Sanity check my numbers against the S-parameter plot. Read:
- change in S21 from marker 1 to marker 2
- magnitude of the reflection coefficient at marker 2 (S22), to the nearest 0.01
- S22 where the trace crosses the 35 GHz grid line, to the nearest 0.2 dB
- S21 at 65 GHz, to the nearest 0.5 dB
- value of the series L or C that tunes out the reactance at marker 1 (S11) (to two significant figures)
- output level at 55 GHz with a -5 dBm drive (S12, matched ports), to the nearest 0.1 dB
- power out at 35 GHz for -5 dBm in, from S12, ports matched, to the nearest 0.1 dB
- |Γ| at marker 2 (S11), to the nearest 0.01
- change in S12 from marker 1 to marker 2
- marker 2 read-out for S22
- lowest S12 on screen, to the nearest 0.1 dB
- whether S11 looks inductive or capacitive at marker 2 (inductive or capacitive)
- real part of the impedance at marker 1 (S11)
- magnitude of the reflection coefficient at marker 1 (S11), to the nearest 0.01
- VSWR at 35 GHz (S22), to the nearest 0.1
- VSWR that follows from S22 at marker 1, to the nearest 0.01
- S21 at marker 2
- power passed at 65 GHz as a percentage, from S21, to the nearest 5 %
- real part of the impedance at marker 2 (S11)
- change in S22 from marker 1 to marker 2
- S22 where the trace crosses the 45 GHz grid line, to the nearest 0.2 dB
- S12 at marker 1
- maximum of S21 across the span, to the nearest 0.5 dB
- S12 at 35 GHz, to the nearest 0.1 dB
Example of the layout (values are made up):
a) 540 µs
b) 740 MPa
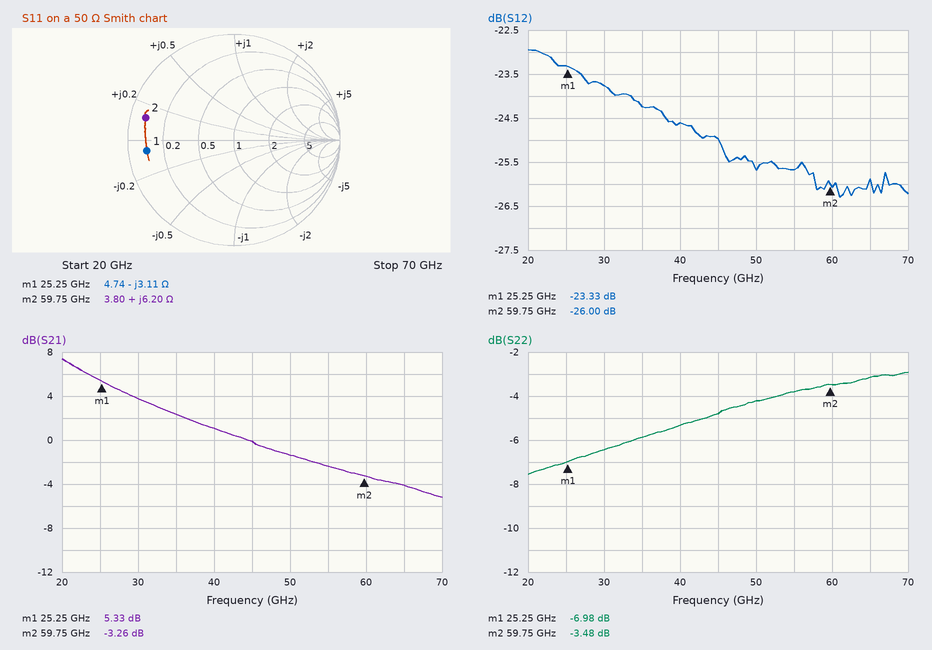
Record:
a) -8.59 dB
b) 0.67
c) -5.8 dB
d) -4.0 dB
e) 20 pH
f) -30.7 dBm
g) -29.2 dBm
h) 0.86
i) -2.67 dB
j) -3.48 dB
k) -26.3 dB
l) inductive
m) 4.74 Ω
n) 0.83
o) 3.1
p) 2.62
q) -3.26 dB
r) 40 %
s) 3.80 Ω
t) 3.50 dB
u) -4.8 dB
v) -23.33 dB
w) 7.5 dB
x) -24.2 dB
